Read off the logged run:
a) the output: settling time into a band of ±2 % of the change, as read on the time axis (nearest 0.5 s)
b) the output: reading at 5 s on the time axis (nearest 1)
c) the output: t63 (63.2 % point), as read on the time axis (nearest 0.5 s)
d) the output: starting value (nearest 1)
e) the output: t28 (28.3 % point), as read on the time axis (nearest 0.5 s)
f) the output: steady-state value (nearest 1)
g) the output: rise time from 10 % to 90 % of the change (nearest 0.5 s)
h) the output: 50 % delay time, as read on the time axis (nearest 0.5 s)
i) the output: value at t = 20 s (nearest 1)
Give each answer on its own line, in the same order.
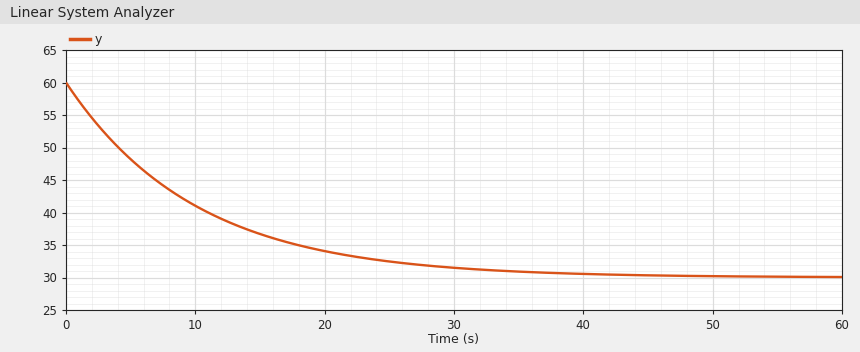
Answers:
39.0 s
48
10.0 s
60
3.5 s
30
22.0 s
7.0 s
34
